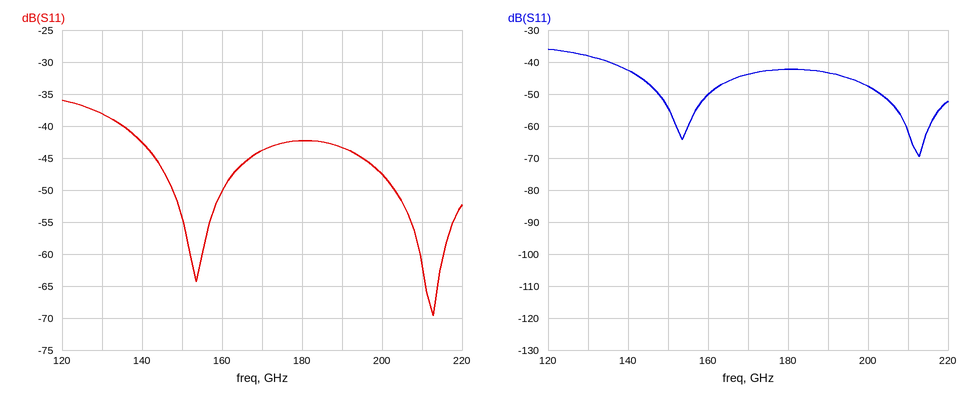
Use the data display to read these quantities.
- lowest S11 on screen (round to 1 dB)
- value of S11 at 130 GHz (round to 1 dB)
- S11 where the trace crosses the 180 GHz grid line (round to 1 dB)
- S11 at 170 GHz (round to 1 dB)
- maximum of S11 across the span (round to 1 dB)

-70 dB
-38 dB
-42 dB
-44 dB
-36 dB
